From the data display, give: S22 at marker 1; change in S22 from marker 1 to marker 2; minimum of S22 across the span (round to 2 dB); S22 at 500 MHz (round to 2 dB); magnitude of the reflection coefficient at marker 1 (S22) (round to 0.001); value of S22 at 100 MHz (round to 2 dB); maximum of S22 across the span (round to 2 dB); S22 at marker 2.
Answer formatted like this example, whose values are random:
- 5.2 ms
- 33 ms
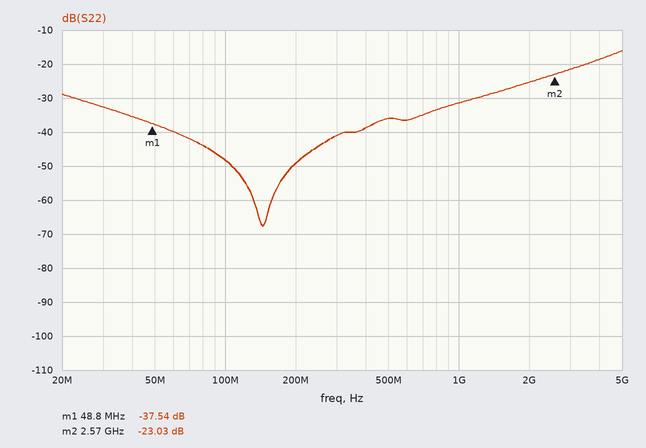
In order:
- -37.54 dB
- 14.51 dB
- -68 dB
- -36 dB
- 0.013
- -48 dB
- -16 dB
- -23.03 dB
